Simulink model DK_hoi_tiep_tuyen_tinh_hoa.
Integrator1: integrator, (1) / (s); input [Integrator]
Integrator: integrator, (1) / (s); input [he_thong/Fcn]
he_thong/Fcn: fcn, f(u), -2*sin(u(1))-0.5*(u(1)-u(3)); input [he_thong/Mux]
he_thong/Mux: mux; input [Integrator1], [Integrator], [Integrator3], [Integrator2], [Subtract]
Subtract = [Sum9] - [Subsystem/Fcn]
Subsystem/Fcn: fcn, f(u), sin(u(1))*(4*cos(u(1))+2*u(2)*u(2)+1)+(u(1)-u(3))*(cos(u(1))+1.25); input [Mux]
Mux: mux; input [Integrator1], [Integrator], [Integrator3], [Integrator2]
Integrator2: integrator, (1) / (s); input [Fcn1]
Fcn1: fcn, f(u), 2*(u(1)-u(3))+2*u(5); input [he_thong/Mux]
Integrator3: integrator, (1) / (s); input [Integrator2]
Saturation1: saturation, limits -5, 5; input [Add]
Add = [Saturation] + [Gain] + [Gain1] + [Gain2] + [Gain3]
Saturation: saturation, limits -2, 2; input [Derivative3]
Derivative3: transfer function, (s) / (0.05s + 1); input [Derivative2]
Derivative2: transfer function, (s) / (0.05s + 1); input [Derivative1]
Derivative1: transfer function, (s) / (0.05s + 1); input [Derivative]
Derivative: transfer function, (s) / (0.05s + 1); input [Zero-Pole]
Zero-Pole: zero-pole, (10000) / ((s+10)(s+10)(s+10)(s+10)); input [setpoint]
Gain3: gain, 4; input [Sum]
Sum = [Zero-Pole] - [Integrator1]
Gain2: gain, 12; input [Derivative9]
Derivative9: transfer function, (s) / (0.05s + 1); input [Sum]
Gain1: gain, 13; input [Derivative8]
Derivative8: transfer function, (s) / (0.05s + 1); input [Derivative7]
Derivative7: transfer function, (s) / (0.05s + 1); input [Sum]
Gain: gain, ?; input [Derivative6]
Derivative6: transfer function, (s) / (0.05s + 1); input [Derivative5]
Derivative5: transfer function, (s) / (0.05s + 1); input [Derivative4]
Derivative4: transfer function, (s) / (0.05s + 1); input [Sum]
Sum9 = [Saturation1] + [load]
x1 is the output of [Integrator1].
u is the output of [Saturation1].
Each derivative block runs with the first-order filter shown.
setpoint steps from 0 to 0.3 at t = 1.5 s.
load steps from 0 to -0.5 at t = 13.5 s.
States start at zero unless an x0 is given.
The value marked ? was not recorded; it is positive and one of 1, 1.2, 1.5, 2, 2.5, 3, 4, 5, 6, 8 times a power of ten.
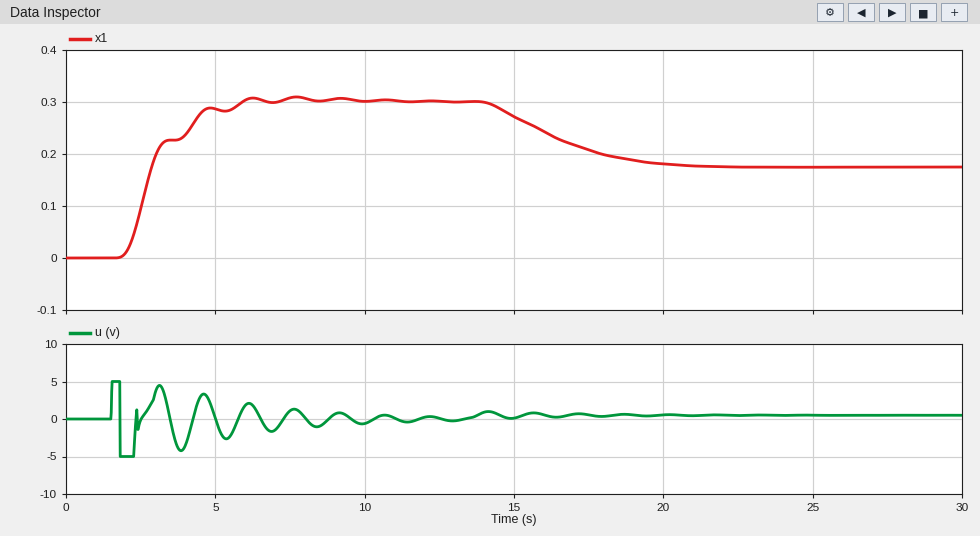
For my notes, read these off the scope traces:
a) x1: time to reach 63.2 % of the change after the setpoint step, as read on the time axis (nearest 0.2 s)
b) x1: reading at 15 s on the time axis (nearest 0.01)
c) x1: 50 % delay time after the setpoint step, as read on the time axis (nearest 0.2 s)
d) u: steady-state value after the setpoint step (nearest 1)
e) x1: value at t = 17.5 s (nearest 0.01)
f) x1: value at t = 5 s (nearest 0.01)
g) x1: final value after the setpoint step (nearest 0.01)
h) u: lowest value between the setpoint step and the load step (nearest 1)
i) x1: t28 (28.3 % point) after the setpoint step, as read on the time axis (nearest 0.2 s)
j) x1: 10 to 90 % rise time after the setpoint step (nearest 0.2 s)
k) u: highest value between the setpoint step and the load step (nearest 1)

3.0 s
0.27
2.8 s
0
0.21
0.29
0.30
-5
2.4 s
2.2 s
5
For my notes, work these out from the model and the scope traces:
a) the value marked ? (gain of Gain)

3
